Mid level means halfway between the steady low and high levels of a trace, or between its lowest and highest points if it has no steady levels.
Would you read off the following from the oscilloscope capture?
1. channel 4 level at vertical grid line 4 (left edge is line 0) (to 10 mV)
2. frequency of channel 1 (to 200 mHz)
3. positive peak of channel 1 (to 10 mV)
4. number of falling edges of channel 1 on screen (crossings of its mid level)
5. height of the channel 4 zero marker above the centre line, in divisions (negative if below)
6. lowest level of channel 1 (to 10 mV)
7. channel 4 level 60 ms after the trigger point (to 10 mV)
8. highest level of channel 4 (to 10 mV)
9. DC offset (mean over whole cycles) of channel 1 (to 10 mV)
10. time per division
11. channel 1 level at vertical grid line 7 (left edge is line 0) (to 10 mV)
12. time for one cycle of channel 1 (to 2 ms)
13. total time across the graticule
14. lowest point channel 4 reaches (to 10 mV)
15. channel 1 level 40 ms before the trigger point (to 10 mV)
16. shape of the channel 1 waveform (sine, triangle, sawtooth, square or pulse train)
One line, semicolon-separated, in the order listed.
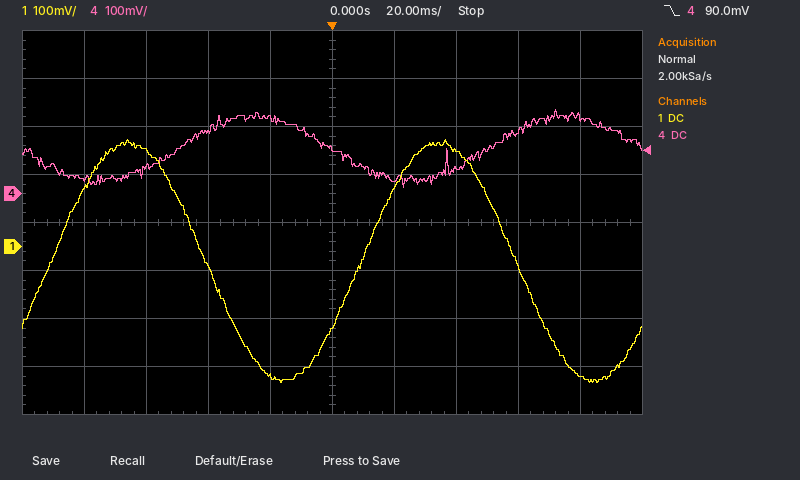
160 mV; 10.0 Hz; 220 mV; 2; +0.6 div; -280 mV; 130 mV; 180 mV; -30 mV; 20 ms; 200 mV; 100 ms; 200 ms; 10 mV; -40 mV; sine
